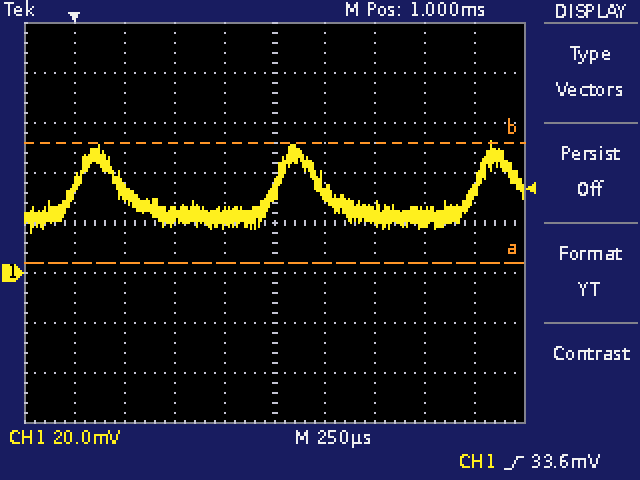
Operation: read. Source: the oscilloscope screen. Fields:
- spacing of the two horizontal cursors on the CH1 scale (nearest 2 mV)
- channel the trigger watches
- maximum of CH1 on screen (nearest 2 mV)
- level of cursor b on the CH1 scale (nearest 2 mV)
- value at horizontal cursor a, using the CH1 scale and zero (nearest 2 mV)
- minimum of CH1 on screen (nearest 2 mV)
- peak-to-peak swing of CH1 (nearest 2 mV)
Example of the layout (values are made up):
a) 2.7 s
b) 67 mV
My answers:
a) 48 mV
b) CH1
c) 52 mV
d) 52 mV
e) 4 mV
f) 16 mV
g) 36 mV
